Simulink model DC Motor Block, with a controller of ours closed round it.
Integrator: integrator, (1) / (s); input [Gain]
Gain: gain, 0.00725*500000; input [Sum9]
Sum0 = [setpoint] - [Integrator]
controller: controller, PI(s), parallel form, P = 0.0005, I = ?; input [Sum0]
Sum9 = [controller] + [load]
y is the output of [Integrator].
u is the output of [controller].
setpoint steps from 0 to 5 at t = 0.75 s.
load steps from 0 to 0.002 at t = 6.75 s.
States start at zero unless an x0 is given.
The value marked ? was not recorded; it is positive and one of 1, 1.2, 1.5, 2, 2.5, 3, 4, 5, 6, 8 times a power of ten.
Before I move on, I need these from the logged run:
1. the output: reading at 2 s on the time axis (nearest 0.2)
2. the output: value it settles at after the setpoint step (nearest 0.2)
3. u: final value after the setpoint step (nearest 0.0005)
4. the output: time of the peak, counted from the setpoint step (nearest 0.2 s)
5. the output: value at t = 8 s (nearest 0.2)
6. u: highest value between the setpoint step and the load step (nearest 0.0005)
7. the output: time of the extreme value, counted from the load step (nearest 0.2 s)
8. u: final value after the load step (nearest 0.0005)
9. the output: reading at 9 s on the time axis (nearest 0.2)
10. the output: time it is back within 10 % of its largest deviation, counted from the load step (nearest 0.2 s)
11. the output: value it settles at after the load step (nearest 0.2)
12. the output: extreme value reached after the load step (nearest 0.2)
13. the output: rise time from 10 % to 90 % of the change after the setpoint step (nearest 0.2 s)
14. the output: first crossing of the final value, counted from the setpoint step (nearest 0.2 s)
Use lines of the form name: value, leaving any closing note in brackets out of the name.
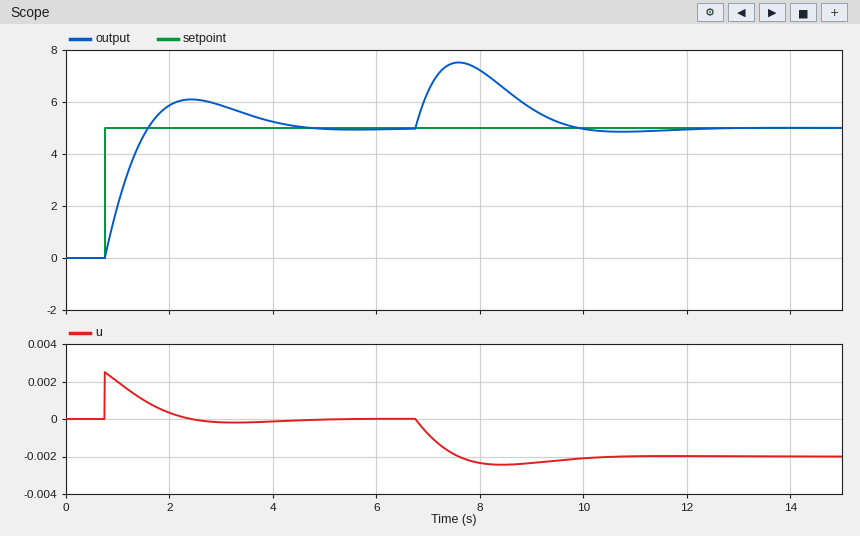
the output: reading at 2 s on the time axis: 5.8
the output: value it settles at after the setpoint step: 5.0
u: final value after the setpoint step: 0.0000
the output: time of the peak, counted from the setpoint step: 1.6 s
the output: value at t = 8 s: 7.2
u: highest value between the setpoint step and the load step: 0.0025
the output: time of the extreme value, counted from the load step: 0.8 s
u: final value after the load step: -0.0020
the output: reading at 9 s on the time axis: 5.8
the output: time it is back within 10 % of its largest deviation, counted from the load step: 2.8 s
the output: value it settles at after the load step: 5.0
the output: extreme value reached after the load step: 7.6
the output: rise time from 10 % to 90 % of the change after the setpoint step: 0.6 s
the output: first crossing of the final value, counted from the setpoint step: 0.8 s
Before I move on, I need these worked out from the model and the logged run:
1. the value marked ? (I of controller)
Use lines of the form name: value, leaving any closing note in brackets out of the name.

the value marked ?: 0.0005
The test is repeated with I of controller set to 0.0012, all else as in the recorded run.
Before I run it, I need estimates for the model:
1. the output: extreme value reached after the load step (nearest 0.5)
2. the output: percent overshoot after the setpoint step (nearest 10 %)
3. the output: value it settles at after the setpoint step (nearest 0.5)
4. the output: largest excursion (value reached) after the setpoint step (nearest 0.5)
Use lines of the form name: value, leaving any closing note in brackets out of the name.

the output: extreme value reached after the load step: 7.0
the output: percent overshoot after the setpoint step: 30 %
the output: value it settles at after the setpoint step: 5.0
the output: largest excursion (value reached) after the setpoint step: 6.5
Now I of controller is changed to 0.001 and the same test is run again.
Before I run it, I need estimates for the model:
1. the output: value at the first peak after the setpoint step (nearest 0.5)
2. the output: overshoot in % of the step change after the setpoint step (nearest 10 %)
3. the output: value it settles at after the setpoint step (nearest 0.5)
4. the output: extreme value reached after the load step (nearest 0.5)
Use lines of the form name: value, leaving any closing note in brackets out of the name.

the output: value at the first peak after the setpoint step: 6.5
the output: overshoot in % of the step change after the setpoint step: 30 %
the output: value it settles at after the setpoint step: 5.0
the output: extreme value reached after the load step: 7.0
